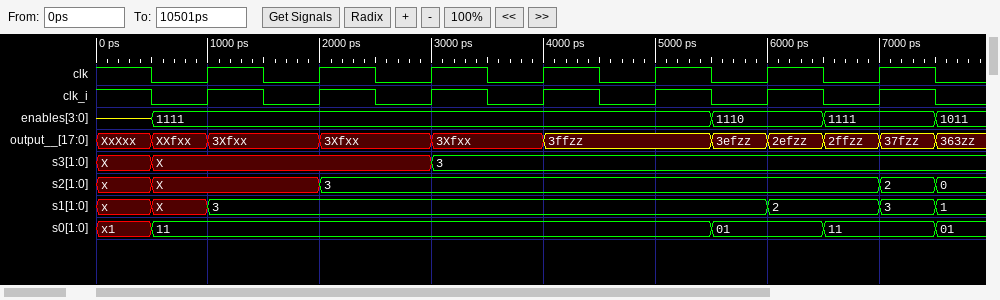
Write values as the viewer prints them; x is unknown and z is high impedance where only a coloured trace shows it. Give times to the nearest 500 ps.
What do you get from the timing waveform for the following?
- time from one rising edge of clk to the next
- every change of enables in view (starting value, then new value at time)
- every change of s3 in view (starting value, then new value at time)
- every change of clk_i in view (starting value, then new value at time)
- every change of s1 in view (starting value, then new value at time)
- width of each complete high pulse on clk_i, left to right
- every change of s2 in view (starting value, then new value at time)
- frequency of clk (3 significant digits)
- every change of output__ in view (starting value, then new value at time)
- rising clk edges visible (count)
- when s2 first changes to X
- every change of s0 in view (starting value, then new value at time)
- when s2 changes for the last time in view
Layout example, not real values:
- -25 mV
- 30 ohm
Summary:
- 1000 ps
- z, 1111 at 500 ps, 1110 at 5500 ps, 1111 at 6500 ps, 1011 at 7500 ps
- X, X at 500 ps, 3 at 3000 ps
- 1, 0 at 500 ps, 1 at 1000 ps, 0 at 1500 ps, 1 at 2000 ps, 0 at 2500 ps, 1 at 3000 ps, 0 at 3500 ps, 1 at 4000 ps, 0 at 4500 ps, 1 at 5000 ps, 0 at 5500 ps, 1 at 6000 ps, 0 at 6500 ps, 1 at 7000 ps, 0 at 7500 ps
- x, X at 500 ps, 3 at 1000 ps, 2 at 6000 ps, 3 at 7000 ps, 1 at 7500 ps
- 500 ps, 500 ps, 500 ps, 500 ps, 500 ps, 500 ps, 500 ps
- x, X at 500 ps, 3 at 2000 ps, 2 at 7000 ps, 0 at 7500 ps
- 1.00 GHz
- XxXxx, XXfxx at 500 ps, 3Xfxx at 1000 ps, 3Xfxx at 2000 ps, 3Xfxx at 3000 ps, 3ffzz at 4000 ps, 3efzz at 5500 ps, 2efzz at 6000 ps, 2ffzz at 6500 ps, 37fzz at 7000 ps, 363zz at 7500 ps
- 7
- 500 ps
- x1, 11 at 500 ps, 01 at 5500 ps, 11 at 6500 ps, 01 at 7500 ps
- 7500 ps
